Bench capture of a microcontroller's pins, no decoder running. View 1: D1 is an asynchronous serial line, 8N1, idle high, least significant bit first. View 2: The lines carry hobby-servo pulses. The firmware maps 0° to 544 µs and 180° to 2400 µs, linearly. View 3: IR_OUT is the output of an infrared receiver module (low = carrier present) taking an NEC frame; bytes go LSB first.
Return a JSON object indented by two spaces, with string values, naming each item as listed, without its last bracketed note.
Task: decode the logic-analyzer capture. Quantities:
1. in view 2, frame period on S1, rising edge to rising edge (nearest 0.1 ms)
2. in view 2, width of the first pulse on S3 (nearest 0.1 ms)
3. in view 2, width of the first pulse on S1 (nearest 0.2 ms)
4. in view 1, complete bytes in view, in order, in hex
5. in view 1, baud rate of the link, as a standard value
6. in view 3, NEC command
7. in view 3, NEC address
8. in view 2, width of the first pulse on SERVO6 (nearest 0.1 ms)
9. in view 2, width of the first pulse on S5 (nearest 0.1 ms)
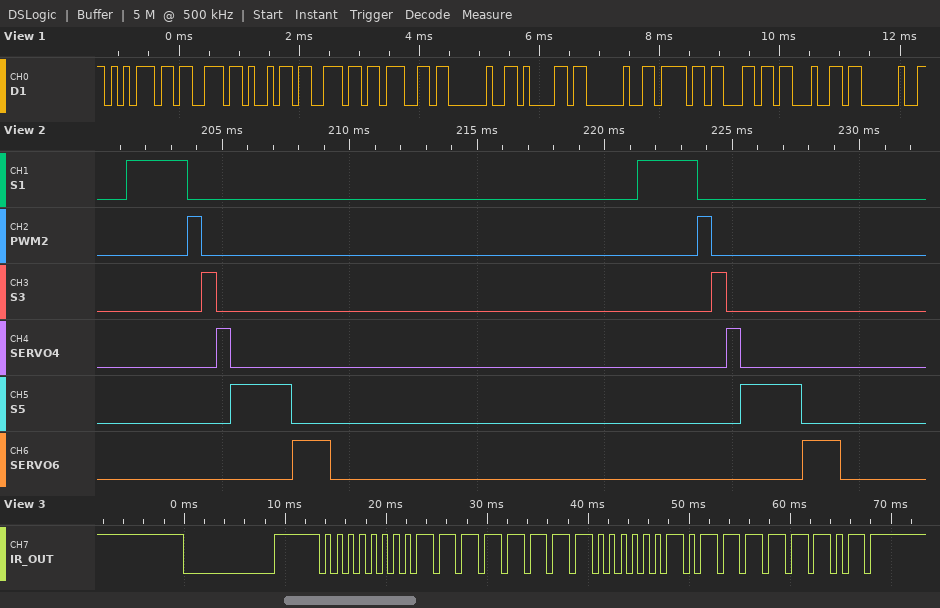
{
  "in view 2, frame period on S1, rising edge to rising edge": "20.0 ms",
  "in view 2, width of the first pulse on S3": "0.6 ms",
  "in view 2, width of the first pulse on S1": "2.4 ms",
  "in view 1, complete bytes in view, in order, in hex": "0x75 0x73 0x69 0x6E 0x67 0x20 0x61 0x20 0x6F 0x6C 0x64 0x20",
  "in view 1, baud rate of the link, as a standard value": "9600 baud",
  "in view 3, NEC command": "0x40",
  "in view 3, NEC address": "0x00",
  "in view 2, width of the first pulse on SERVO6": "1.5 ms",
  "in view 2, width of the first pulse on S5": "2.4 ms"
}
